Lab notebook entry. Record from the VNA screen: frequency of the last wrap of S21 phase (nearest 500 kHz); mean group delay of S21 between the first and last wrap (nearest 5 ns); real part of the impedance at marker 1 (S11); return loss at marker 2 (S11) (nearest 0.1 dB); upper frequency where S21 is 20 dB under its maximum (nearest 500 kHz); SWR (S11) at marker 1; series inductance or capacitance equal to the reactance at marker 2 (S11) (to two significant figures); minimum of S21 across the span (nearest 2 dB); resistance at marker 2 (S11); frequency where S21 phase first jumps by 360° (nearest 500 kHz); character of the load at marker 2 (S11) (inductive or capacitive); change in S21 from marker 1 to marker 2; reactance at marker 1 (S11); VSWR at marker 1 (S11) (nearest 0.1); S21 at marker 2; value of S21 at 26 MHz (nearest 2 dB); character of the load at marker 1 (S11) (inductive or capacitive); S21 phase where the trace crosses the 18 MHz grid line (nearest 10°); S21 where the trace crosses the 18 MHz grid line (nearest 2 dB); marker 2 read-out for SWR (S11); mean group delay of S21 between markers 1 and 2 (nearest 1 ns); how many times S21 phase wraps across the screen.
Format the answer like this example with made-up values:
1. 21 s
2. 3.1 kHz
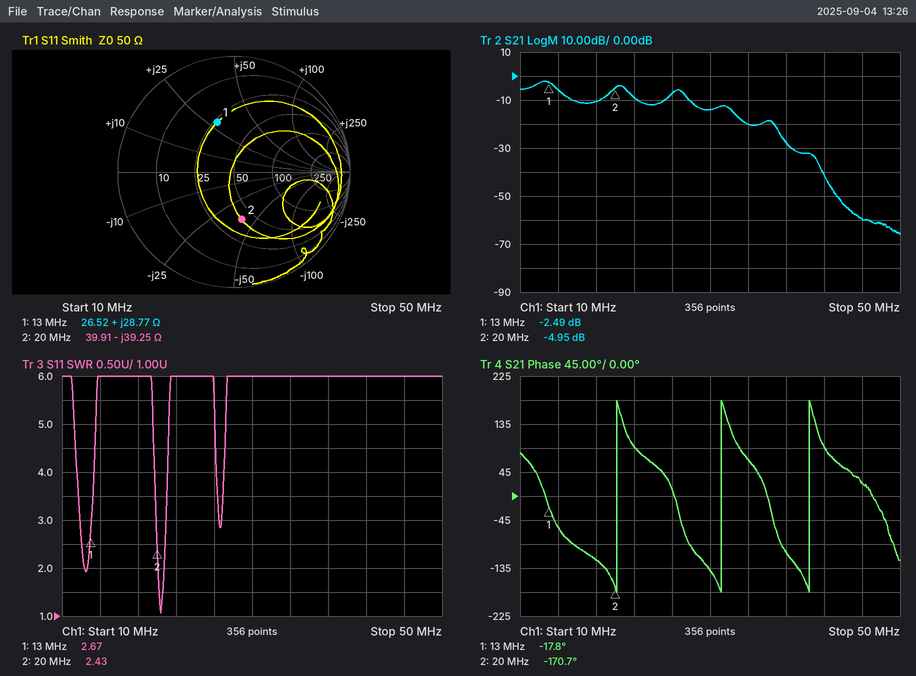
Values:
1. 40.5 MHz
2. 100 ns
3. 26.52 Ω
4. 7.7 dB
5. 37.0 MHz
6. 2.67
7. 200 pF
8. -66 dB
9. 39.91 Ω
10. 20.0 MHz
11. capacitive
12. -2.46 dB
13. +28.77 Ω
14. 2.7
15. -4.95 dB
16. -8 dB
17. inductive
18. -120°
19. -10 dB
20. 2.43
21. 61 ns
22. 3
